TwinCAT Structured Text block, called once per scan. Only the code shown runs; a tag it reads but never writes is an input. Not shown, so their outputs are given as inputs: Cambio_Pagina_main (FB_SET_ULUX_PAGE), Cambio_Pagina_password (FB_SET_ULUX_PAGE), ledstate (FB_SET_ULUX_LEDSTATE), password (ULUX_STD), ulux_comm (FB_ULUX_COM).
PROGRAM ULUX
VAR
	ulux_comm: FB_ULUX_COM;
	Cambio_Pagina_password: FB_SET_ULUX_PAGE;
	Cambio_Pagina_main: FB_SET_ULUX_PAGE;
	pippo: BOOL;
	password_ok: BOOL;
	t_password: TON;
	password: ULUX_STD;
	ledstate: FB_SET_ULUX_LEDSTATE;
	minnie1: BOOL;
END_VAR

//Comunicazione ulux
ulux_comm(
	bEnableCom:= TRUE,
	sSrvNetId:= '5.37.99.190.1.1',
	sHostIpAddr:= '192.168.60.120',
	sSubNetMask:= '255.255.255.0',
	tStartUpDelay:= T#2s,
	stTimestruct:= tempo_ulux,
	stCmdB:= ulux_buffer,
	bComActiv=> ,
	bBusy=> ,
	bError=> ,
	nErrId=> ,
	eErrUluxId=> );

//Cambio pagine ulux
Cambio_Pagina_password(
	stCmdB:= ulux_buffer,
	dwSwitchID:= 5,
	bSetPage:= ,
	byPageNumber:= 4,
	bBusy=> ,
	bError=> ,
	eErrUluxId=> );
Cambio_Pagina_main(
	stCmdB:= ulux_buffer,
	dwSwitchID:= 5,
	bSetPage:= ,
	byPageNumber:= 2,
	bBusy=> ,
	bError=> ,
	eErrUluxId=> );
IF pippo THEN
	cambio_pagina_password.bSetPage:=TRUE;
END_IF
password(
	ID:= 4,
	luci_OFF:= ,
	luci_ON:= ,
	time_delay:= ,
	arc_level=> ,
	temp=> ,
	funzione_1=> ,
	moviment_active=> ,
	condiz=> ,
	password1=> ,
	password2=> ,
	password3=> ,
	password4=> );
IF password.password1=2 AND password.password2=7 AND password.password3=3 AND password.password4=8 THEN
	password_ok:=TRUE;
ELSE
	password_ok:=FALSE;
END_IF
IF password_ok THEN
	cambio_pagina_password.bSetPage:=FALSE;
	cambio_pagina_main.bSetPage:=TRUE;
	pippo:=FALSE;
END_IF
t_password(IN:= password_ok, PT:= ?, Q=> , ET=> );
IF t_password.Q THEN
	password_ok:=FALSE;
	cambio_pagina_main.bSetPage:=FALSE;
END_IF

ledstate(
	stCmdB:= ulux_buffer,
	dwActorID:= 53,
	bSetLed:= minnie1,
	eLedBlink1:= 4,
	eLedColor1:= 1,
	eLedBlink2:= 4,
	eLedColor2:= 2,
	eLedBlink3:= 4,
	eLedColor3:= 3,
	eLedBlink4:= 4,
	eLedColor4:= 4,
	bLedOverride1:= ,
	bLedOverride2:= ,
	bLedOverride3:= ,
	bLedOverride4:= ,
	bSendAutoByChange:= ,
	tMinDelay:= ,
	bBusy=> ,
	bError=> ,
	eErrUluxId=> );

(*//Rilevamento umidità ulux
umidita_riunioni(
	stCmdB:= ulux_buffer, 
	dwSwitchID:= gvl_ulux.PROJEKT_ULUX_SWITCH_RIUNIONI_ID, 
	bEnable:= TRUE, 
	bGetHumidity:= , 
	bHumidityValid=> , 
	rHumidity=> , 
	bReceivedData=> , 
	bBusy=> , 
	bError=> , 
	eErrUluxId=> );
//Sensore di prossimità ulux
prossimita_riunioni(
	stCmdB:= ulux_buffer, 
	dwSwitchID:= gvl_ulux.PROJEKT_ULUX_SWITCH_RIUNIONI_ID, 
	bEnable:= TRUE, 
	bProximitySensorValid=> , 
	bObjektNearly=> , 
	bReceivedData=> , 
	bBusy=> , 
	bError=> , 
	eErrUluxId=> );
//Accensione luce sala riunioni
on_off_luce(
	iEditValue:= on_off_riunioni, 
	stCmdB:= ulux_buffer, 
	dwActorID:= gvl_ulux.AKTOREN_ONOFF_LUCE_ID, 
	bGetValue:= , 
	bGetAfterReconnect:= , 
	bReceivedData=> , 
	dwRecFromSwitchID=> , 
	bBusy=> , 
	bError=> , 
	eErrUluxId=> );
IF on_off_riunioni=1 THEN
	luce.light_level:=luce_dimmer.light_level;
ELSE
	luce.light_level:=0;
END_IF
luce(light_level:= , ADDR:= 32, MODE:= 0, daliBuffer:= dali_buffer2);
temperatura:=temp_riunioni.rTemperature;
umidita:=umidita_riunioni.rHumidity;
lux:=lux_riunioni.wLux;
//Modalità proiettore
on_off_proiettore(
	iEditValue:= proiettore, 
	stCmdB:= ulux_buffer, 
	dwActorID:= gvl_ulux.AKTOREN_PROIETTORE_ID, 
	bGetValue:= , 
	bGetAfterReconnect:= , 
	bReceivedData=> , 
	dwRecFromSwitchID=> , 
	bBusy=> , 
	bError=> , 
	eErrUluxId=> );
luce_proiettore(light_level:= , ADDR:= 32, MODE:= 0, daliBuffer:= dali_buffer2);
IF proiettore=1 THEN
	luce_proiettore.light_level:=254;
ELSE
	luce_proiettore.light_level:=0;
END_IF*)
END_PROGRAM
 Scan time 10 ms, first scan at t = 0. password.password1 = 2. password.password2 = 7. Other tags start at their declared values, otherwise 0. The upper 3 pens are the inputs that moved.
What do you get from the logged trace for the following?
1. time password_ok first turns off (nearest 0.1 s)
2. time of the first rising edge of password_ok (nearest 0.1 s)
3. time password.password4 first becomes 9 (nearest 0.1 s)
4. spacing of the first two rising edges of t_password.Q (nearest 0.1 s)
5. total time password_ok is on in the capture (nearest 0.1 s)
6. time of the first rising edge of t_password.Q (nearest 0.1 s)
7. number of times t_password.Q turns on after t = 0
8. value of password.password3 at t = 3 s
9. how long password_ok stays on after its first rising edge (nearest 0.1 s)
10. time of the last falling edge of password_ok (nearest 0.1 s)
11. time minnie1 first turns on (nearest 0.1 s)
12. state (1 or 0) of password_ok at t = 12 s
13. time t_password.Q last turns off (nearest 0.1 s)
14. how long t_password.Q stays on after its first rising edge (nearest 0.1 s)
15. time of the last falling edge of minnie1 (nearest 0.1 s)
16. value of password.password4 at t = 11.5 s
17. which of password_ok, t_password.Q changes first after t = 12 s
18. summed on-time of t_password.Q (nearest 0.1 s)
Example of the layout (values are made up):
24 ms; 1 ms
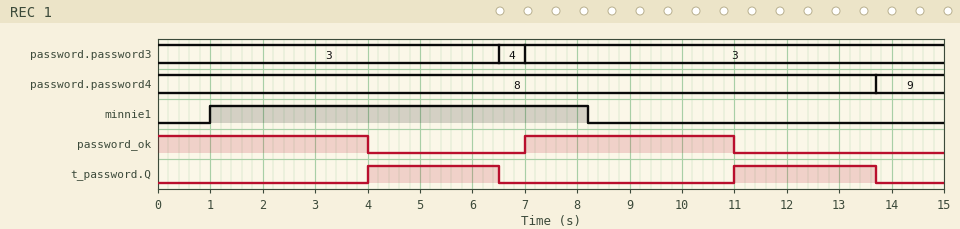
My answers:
4.0 s; 7.0 s; 13.7 s; 7.0 s; 8.0 s; 4.0 s; 2; 3; 4.0 s; 11.0 s; 1.0 s; 0; 13.7 s; 2.5 s; 8.2 s; 8; t_password.Q; 5.2 s
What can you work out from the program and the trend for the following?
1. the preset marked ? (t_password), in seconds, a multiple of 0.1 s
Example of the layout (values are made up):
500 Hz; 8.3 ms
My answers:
4.0 s
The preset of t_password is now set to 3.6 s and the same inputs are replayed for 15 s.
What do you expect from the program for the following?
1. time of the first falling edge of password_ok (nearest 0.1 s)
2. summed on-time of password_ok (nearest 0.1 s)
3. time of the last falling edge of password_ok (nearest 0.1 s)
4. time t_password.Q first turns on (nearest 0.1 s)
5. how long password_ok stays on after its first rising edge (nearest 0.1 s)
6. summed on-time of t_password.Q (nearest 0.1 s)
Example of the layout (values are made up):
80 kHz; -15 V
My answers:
3.6 s; 7.2 s; 10.6 s; 3.6 s; 3.6 s; 6.0 s
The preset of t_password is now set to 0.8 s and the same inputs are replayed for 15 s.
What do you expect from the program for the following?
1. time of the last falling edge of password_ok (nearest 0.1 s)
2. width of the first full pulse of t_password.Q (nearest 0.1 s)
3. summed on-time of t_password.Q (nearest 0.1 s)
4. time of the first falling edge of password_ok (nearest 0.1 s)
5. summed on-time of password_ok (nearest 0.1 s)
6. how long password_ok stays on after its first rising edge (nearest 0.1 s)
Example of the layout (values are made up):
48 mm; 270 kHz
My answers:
7.8 s; 5.7 s; 11.6 s; 0.8 s; 1.6 s; 0.8 s
